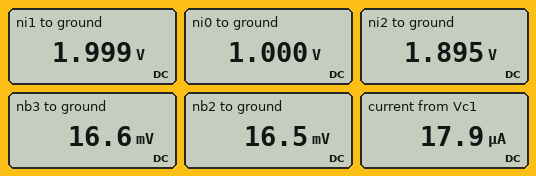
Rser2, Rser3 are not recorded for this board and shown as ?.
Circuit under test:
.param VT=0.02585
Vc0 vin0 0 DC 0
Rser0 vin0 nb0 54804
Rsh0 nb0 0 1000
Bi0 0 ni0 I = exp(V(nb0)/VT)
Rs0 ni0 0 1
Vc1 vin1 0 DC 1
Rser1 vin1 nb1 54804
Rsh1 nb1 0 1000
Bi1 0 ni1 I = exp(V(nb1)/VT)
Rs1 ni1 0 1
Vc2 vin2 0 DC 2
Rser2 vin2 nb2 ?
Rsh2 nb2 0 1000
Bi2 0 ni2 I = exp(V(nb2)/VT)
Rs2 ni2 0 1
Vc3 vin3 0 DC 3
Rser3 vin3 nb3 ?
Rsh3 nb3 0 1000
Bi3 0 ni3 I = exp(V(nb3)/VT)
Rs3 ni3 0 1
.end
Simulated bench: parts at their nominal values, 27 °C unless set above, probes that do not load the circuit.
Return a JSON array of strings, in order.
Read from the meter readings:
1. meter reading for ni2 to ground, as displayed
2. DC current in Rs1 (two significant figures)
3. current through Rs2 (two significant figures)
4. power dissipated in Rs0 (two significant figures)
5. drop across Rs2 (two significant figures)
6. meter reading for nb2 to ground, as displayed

["1.895 V", "2.0 A", "1.9 A", "1.0 W", "1.9 V", "16.5 mV"]
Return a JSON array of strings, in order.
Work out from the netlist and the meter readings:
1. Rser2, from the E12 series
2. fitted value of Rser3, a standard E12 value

["120 kΩ", "180 kΩ"]
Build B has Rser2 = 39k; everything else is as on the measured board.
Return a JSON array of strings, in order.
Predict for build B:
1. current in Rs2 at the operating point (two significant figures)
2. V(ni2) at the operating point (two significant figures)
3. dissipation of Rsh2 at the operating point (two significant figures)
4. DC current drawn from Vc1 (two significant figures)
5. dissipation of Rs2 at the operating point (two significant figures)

["6.9 A", "6.9 V", "2.5 µW", "18 µA", "48 W"]
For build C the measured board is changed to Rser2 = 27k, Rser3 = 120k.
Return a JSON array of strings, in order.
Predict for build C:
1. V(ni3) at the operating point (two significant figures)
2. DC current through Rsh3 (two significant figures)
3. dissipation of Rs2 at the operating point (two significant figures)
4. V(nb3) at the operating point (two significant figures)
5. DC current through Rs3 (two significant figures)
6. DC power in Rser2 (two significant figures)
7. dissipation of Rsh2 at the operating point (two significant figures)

["2.6 V", "25 µA", "250 W", "25 mV", "2.6 A", "140 µW", "5.1 µW"]
